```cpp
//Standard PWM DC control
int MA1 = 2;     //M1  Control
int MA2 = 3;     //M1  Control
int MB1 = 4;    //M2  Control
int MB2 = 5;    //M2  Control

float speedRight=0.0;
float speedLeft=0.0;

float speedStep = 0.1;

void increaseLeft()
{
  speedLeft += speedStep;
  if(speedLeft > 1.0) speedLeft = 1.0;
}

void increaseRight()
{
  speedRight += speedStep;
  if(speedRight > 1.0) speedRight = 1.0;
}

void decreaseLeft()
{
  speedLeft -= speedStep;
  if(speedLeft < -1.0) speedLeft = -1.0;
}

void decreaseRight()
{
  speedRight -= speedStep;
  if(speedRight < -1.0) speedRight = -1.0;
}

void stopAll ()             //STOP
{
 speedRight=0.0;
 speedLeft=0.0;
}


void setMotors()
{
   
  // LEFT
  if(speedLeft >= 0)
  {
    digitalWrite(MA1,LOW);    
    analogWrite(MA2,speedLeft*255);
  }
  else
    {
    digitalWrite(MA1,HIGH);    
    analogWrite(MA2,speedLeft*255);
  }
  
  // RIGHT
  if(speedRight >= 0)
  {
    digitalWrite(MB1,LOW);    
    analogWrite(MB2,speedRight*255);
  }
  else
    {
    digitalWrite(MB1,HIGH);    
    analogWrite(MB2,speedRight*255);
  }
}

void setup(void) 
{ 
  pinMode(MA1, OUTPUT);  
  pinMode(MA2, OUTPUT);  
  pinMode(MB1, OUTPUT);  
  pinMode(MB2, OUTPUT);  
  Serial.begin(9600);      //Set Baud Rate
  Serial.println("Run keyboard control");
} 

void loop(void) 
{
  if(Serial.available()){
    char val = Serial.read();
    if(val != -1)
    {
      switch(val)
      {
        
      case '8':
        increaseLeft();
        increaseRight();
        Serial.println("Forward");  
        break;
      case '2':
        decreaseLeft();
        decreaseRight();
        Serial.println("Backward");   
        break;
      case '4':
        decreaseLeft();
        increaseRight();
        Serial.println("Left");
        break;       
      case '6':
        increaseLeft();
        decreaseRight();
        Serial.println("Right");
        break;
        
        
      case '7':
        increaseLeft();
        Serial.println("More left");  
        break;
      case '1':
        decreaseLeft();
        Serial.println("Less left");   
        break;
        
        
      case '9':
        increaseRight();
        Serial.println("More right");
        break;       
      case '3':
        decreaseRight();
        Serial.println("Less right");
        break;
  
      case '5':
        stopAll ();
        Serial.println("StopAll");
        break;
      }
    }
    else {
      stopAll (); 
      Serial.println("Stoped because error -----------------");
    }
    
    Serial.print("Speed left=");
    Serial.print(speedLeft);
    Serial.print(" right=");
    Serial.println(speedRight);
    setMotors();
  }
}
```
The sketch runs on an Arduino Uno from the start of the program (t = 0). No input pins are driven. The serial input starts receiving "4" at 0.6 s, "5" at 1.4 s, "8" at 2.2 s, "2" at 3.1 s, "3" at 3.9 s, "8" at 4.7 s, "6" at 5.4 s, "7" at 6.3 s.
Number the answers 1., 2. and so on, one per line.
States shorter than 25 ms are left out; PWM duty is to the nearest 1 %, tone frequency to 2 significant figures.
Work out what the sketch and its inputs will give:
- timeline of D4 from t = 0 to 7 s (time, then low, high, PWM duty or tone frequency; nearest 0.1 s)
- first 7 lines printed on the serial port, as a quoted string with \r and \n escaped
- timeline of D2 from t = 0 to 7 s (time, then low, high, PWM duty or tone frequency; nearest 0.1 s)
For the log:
1. 0 s low; 3.9 s high; 4.7 s low; 5.4 s high
2. "Run keyboard control\r\nLeft\r\nSpeed left=-0.10 right=0.10\r\nStopAll\r\nSpeed left=0.00 right=0.00\r\nForward\r\nSpeed left=0.10 right=0.10\r\n"
3. 0 s low; 0.6 s high; 1.4 s low
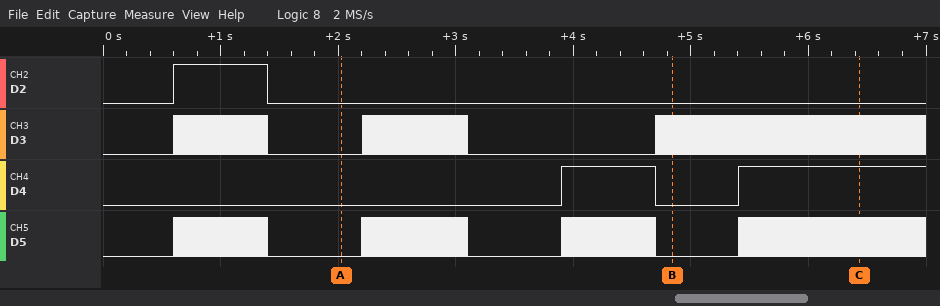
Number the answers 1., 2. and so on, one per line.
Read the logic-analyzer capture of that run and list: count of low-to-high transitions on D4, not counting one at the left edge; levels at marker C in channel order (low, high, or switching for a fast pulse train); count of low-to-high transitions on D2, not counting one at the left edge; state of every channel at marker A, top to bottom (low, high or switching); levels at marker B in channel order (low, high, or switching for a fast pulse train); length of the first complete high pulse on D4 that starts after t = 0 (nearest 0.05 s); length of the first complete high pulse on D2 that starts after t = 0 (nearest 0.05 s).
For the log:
1. 2
2. D2 low, D3 switching, D4 high, D5 switching
3. 1
4. D2 low, D3 low, D4 low, D5 low
5. D2 low, D3 switching, D4 low, D5 low
6. 0.80 s
7. 0.80 s
